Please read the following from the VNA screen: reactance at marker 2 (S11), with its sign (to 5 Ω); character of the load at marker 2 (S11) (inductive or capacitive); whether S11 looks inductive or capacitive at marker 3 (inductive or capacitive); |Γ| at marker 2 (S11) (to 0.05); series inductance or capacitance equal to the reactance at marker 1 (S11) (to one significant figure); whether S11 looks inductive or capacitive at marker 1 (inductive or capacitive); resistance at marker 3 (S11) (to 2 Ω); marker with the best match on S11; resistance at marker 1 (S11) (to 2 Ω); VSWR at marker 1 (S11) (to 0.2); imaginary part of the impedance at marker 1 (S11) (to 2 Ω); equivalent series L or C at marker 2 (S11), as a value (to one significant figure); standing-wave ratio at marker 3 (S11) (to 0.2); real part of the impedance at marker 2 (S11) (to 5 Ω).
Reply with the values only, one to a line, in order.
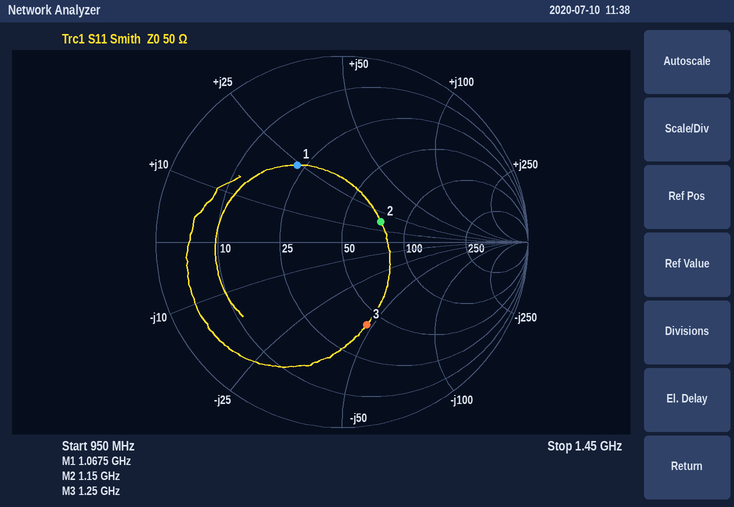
+15 Ω
inductive
capacitive
0.25
4 nH
inductive
42 Ω
marker 2
22 Ω
2.8
+24 Ω
2 nH
2.8
75 Ω
